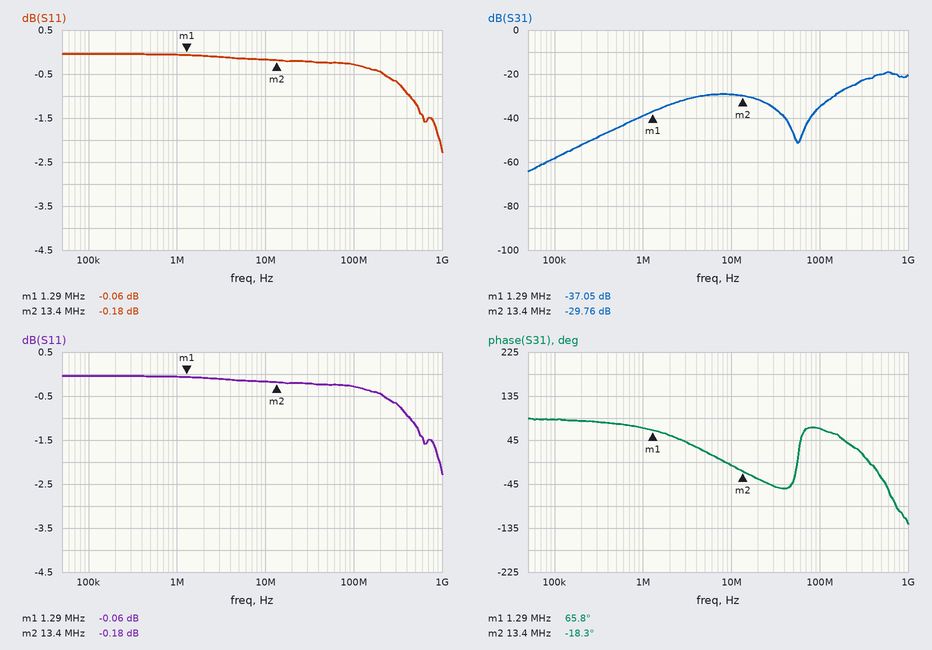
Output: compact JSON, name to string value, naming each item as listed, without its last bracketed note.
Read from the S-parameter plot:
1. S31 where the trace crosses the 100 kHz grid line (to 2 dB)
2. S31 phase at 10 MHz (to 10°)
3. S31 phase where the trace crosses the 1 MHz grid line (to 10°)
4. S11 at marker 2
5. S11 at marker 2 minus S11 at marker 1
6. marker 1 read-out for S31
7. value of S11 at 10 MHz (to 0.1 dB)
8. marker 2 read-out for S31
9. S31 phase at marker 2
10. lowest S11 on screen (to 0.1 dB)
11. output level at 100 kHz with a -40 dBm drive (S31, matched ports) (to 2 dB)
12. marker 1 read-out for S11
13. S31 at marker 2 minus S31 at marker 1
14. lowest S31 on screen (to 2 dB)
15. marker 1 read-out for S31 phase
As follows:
{"S31 where the trace crosses the 100 kHz grid line": "-58 dB", "S31 phase at 10 MHz": "-10°", "S31 phase where the trace crosses the 1 MHz grid line": "70°", "S11 at marker 2": "-0.18 dB", "S11 at marker 2 minus S11 at marker 1": "-0.12 dB", "marker 1 read-out for S31": "-37.05 dB", "value of S11 at 10 MHz": "-0.2 dB", "marker 2 read-out for S31": "-29.76 dB", "S31 phase at marker 2": "-18.3°", "lowest S11 on screen": "-2.3 dB", "output level at 100 kHz with a -40 dBm drive (S31, matched ports)": "-98 dBm", "marker 1 read-out for S11": "-0.06 dB", "S31 at marker 2 minus S31 at marker 1": "7.29 dB", "lowest S31 on screen": "-64 dB", "marker 1 read-out for S31 phase": "65.8°"}
